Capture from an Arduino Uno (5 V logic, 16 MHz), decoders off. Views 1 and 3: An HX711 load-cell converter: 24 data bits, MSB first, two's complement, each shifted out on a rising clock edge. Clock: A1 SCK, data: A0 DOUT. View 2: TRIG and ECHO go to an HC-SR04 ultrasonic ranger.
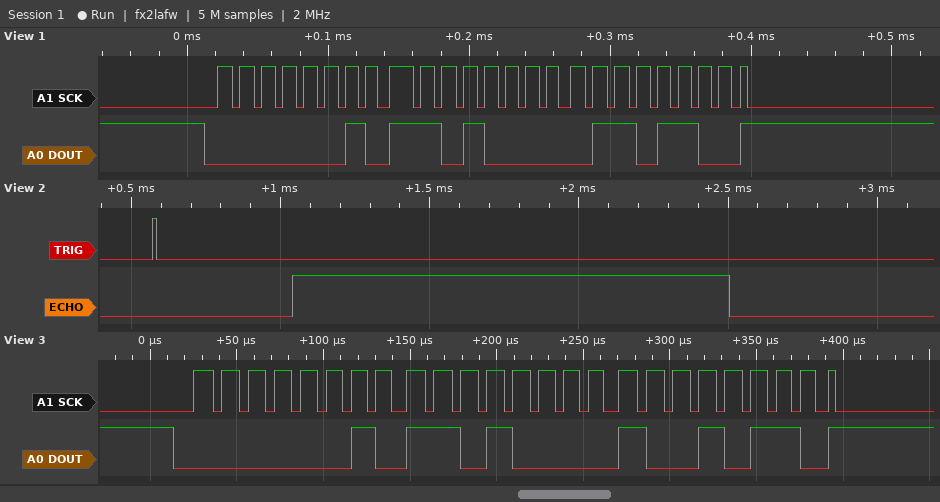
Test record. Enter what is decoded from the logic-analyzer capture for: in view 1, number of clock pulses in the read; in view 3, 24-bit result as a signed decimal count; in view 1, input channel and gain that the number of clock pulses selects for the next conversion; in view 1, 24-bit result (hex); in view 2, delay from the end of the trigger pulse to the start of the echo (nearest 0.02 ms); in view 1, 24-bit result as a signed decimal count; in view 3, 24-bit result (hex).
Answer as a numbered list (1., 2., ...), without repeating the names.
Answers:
1. 25
2. 184470
3. channel A, gain 128
4. 0x02D06C
5. 0.46 ms
6. 184428
7. 0x02D096
